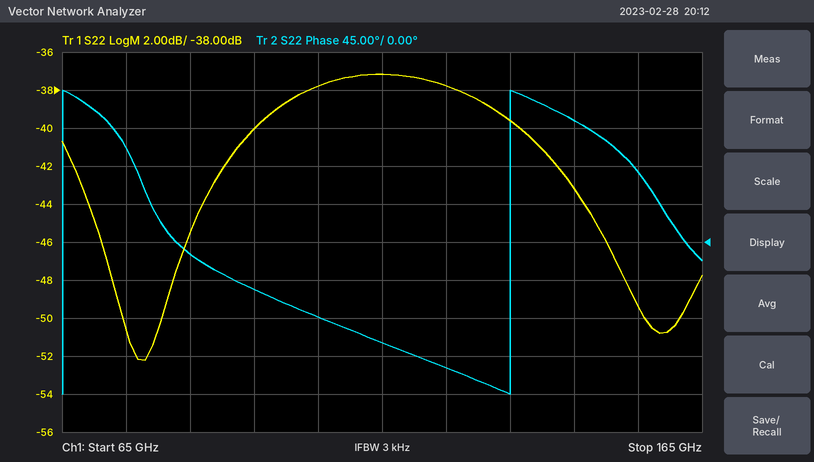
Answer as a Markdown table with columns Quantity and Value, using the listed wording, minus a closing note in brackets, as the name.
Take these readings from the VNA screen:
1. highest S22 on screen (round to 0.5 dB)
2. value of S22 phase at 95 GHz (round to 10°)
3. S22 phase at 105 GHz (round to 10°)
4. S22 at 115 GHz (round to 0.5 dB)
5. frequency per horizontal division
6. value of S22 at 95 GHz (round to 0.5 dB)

| Quantity | Value |
|---|---|
| highest S22 on screen | -37.0 dB |
| value of S22 phase at 95 GHz | -60° |
| S22 phase at 105 GHz | -90° |
| S22 at 115 GHz | -37.0 dB |
| frequency per horizontal division | 10 GHz |
| value of S22 at 95 GHz | -40.0 dB |
